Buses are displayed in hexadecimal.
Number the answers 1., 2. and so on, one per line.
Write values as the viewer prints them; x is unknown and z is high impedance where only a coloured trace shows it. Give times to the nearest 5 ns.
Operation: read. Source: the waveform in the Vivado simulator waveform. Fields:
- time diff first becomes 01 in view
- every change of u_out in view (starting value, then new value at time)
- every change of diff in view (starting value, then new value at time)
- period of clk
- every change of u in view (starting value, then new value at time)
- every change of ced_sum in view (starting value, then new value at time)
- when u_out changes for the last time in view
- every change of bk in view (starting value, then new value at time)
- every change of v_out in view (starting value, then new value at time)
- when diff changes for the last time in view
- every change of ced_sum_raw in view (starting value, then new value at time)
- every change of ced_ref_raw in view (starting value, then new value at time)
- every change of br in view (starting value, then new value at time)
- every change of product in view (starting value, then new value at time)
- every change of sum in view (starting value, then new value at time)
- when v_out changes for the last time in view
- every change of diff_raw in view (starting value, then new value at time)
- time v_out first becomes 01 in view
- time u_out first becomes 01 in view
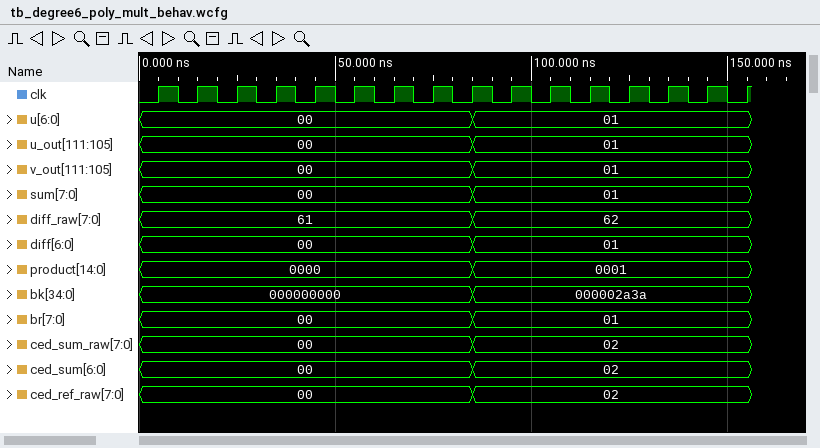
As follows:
1. 85 ns
2. 00, 01 at 85 ns
3. 00, 01 at 85 ns
4. 10 ns
5. 00, 01 at 85 ns
6. 00, 02 at 85 ns
7. 85 ns
8. 000000000, 000002a3a at 85 ns
9. 00, 01 at 85 ns
10. 85 ns
11. 00, 02 at 85 ns
12. 00, 02 at 85 ns
13. 00, 01 at 85 ns
14. 0000, 0001 at 85 ns
15. 00, 01 at 85 ns
16. 85 ns
17. 61, 62 at 85 ns
18. 85 ns
19. 85 ns
